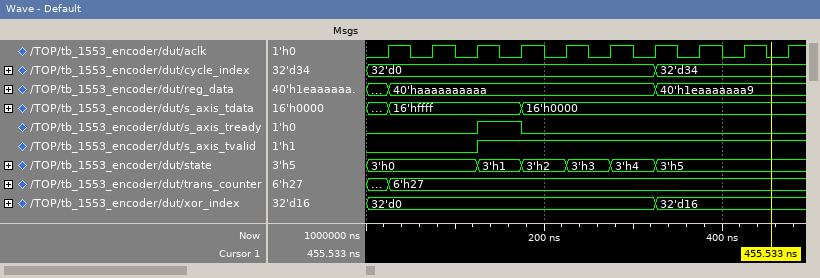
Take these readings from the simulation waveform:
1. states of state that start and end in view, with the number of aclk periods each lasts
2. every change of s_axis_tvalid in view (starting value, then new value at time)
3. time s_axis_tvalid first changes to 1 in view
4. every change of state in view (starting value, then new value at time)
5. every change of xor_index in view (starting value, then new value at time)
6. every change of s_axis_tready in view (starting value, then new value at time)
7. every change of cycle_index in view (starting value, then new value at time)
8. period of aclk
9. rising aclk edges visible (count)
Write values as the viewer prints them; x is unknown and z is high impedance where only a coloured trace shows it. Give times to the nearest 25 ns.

3'h1: 1, 3'h2: 1, 3'h3: 1, 3'h4: 1
0, 1 at 125 ns
125 ns
3'h0, 3'h1 at 125 ns, 3'h2 at 175 ns, 3'h3 at 225 ns, 3'h4 at 275 ns, 3'h5 at 325 ns
32'd0, 32'd16 at 325 ns
0, 1 at 125 ns, 0 at 175 ns
32'd0, 32'd34 at 325 ns
50 ns
10
